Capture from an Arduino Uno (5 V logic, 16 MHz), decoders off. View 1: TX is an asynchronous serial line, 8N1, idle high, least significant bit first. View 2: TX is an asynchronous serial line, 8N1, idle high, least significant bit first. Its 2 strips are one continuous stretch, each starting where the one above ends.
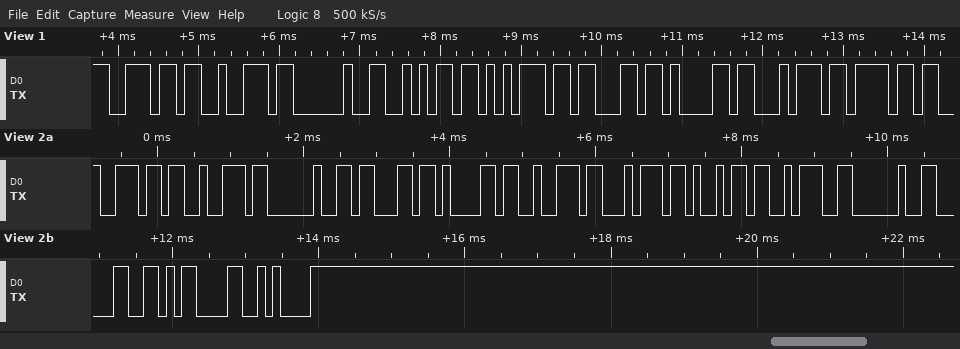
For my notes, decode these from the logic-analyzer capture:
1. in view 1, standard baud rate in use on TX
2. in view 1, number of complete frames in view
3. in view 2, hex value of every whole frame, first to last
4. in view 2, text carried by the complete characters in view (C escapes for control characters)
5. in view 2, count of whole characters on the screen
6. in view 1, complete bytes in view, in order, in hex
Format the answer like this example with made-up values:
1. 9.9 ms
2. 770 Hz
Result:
1. 9600 baud
2. 9
3. 6E 72 20 63 61 72 74 69 3A 20 30 0D 0A
4. "nr carti: 0\r\n"
5. 13
6. 0x6E 0x72 0x20 0x6A 0x75 0x63 0x61 0x74 0x6F
